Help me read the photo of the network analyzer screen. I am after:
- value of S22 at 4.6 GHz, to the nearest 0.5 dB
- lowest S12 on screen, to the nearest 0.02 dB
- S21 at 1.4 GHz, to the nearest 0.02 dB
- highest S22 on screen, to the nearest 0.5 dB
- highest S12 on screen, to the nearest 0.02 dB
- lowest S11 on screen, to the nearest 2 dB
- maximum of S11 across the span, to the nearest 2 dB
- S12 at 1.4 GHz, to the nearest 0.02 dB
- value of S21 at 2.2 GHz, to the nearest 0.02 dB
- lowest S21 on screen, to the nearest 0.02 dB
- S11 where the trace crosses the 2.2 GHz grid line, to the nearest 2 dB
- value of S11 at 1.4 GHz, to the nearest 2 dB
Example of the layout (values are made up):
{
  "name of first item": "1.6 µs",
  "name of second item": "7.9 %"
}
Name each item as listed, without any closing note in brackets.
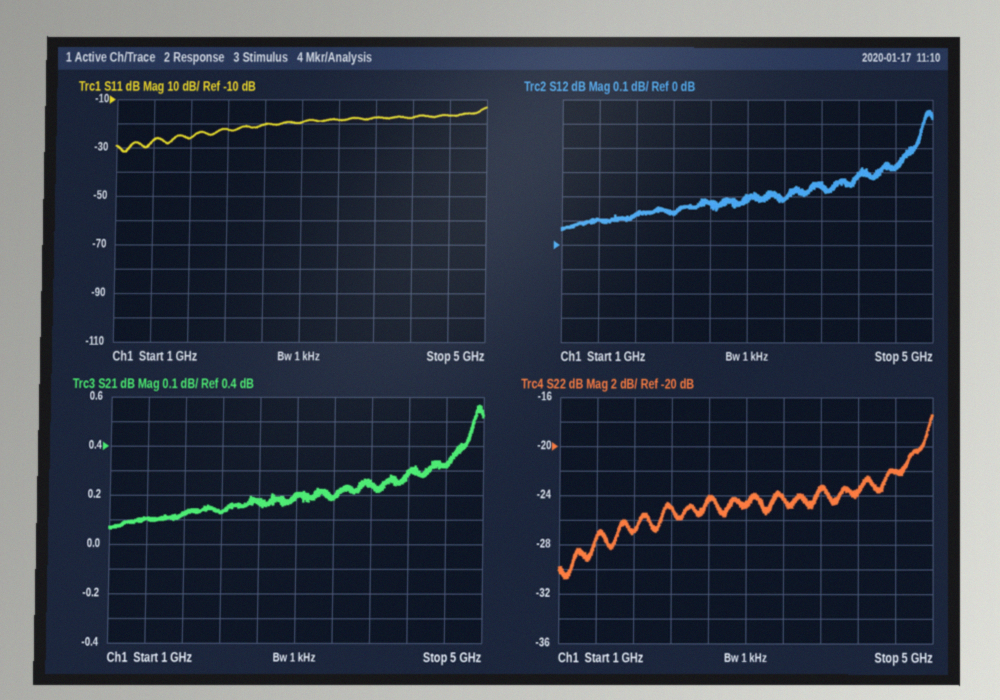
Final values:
{
  "value of S22 at 4.6 GHz, to the nearest 0.5 dB": "-22.0 dB",
  "lowest S12 on screen, to the nearest 0.02 dB": "0.06 dB",
  "S21 at 1.4 GHz, to the nearest 0.02 dB": "0.10 dB",
  "highest S22 on screen, to the nearest 0.5 dB": "-17.5 dB",
  "highest S12 on screen, to the nearest 0.02 dB": "0.56 dB",
  "lowest S11 on screen, to the nearest 2 dB": "-32 dB",
  "maximum of S11 across the span, to the nearest 2 dB": "-14 dB",
  "S12 at 1.4 GHz, to the nearest 0.02 dB": "0.10 dB",
  "value of S21 at 2.2 GHz, to the nearest 0.02 dB": "0.14 dB",
  "lowest S21 on screen, to the nearest 0.02 dB": "0.06 dB",
  "S11 where the trace crosses the 2.2 GHz grid line, to the nearest 2 dB": "-22 dB",
  "value of S11 at 1.4 GHz, to the nearest 2 dB": "-26 dB"
}
